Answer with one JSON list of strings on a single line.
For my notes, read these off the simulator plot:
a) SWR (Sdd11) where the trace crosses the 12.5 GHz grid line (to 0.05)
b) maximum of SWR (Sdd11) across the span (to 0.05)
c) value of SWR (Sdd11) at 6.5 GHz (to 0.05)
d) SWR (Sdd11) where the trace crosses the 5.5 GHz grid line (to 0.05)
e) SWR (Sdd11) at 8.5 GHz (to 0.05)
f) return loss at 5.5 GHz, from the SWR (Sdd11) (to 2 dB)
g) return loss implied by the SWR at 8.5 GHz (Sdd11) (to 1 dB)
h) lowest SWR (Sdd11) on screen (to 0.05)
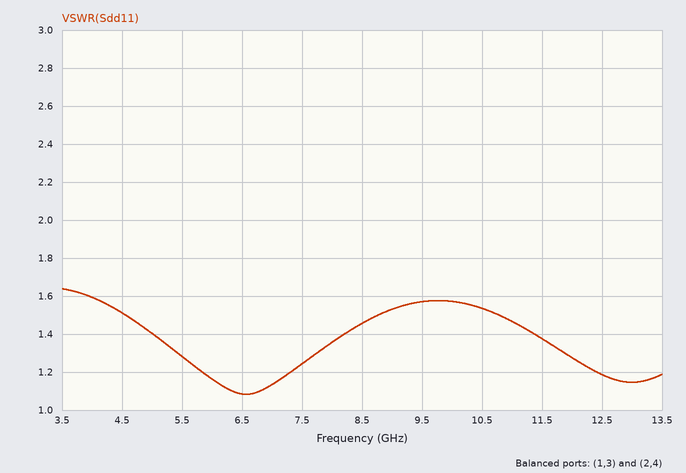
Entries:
["1.20", "1.65", "1.10", "1.30", "1.45", "18 dB", "15 dB", "1.10"]
